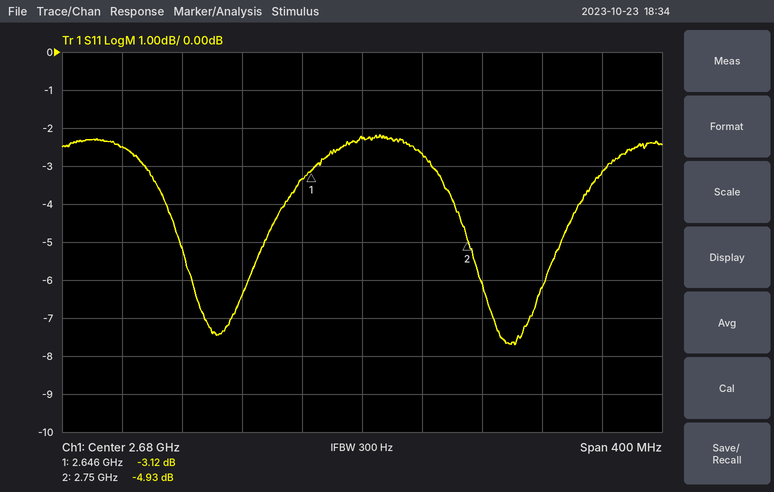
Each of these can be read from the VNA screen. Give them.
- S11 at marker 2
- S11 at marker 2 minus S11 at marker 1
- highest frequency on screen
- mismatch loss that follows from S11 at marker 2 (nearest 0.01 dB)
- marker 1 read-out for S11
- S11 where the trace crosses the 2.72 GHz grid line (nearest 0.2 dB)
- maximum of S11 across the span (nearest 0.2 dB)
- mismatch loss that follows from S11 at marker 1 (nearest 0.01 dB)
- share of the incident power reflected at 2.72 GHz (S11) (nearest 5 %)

-4.93 dB
-1.81 dB
2.88 GHz
1.68 dB
-3.12 dB
-2.6 dB
-2.2 dB
2.90 dB
55 %
